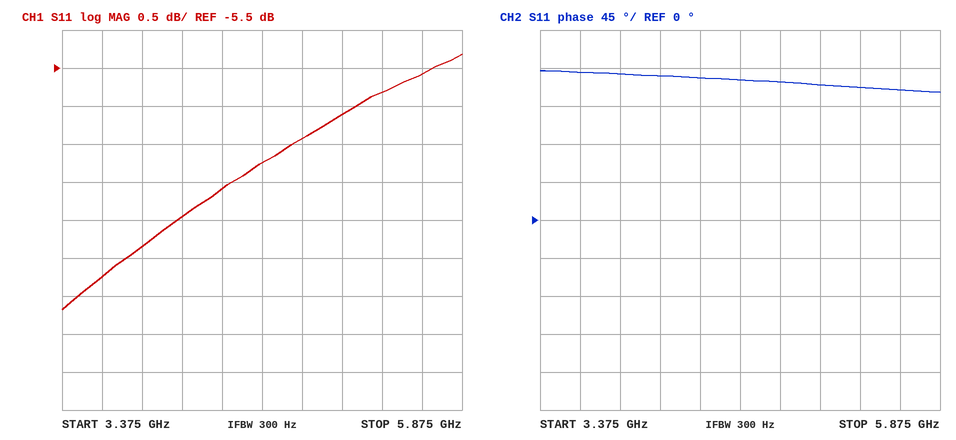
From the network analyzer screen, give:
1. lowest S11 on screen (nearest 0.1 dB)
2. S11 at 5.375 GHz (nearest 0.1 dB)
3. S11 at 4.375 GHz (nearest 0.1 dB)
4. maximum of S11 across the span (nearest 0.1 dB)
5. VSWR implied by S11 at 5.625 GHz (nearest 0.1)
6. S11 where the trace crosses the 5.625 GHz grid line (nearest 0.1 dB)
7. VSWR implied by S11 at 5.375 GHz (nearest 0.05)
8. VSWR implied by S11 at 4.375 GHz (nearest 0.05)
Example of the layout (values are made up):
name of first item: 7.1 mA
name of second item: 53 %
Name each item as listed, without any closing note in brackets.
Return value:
lowest S11 on screen: -8.7 dB
S11 at 5.375 GHz: -5.8 dB
S11 at 4.375 GHz: -7.1 dB
maximum of S11 across the span: -5.3 dB
VSWR implied by S11 at 5.625 GHz: 3.2
S11 where the trace crosses the 5.625 GHz grid line: -5.6 dB
VSWR implied by S11 at 5.375 GHz: 3.10
VSWR implied by S11 at 4.375 GHz: 2.60
